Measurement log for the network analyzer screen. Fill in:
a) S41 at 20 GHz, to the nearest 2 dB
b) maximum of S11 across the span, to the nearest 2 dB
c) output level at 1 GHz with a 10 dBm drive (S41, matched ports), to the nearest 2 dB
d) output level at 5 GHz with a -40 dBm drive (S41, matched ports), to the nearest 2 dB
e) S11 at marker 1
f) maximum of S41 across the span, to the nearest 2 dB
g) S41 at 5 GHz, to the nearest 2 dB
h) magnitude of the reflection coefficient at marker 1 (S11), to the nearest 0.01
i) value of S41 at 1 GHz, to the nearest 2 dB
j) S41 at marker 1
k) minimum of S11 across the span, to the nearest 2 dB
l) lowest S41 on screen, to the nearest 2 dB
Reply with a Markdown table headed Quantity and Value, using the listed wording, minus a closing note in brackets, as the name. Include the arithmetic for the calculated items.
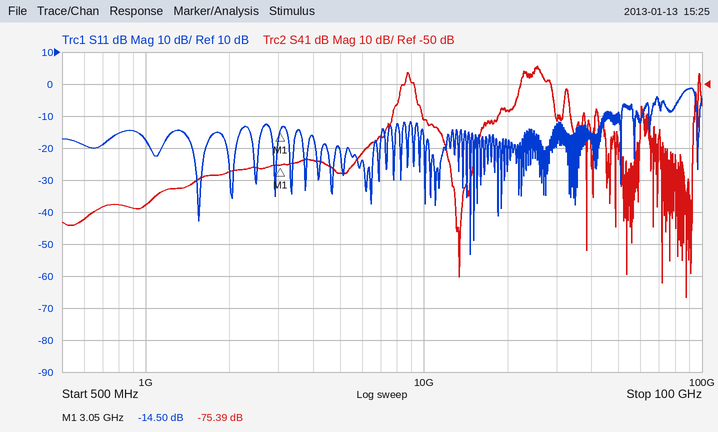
| Quantity | Value |
|---|---|
| S41 at 20 GHz, to the nearest 2 dB | -58 dB |
| maximum of S11 across the span, to the nearest 2 dB | -2 dB |
| output level at 1 GHz with a 10 dBm drive (S41, matched ports), to the nearest 2 dB | 10 dBm + (-88 dB) = -78 dBm |
| output level at 5 GHz with a -40 dBm drive (S41, matched ports), to the nearest 2 dB | -40 dBm + (-78 dB) = -118 dBm |
| S11 at marker 1 | -14.50 dB |
| maximum of S41 across the span, to the nearest 2 dB | -44 dB |
| S41 at 5 GHz, to the nearest 2 dB | -78 dB |
| magnitude of the reflection coefficient at marker 1 (S11), to the nearest 0.01 | 10^(-14.5/20) ≈ 0.19 |
| value of S41 at 1 GHz, to the nearest 2 dB | -88 dB |
| S41 at marker 1 | -75.39 dB |
| minimum of S11 across the span, to the nearest 2 dB | -54 dB |
| lowest S41 on screen, to the nearest 2 dB | -116 dB |
